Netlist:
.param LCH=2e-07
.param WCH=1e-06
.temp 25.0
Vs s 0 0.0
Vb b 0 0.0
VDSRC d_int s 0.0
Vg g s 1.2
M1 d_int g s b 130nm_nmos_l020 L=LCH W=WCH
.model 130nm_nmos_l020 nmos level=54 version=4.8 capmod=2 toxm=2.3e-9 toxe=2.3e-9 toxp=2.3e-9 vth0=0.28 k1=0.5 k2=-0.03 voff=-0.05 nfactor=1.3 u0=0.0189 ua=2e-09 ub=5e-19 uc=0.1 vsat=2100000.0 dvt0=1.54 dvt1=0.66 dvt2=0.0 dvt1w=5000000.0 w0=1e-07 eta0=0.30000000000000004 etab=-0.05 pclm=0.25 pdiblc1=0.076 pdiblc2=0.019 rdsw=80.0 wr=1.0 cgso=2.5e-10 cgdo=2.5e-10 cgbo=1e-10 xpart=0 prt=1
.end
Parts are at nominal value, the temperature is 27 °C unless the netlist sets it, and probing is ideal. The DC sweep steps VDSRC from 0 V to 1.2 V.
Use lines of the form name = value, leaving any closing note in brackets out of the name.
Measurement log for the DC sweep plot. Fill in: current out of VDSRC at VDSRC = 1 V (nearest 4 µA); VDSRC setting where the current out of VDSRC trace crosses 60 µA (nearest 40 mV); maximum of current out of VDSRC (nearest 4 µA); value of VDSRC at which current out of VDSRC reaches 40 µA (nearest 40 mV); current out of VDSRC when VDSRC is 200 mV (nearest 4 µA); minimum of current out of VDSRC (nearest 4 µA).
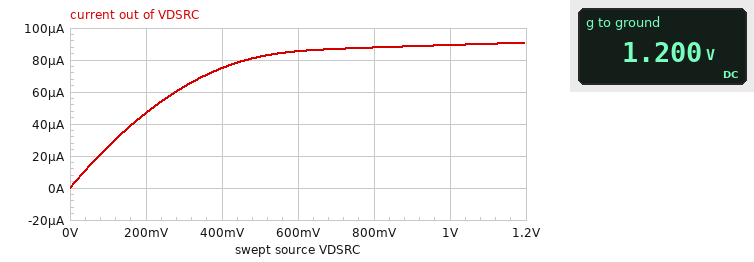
current out of VDSRC at VDSRC = 1 V = 88 µA
VDSRC setting where the current out of VDSRC trace crosses 60 µA = 280 mV
maximum of current out of VDSRC = 92 µA
value of VDSRC at which current out of VDSRC reaches 40 µA = 160 mV
current out of VDSRC when VDSRC is 200 mV = 48 µA
minimum of current out of VDSRC = 0 A
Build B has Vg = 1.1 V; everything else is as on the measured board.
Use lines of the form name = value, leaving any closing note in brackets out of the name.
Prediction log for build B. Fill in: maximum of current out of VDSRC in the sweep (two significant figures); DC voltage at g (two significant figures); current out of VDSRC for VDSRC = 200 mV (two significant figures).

maximum of current out of VDSRC in the sweep = 69 µA
DC voltage at g = 1.1 V
current out of VDSRC for VDSRC = 200 mV = 39 µA
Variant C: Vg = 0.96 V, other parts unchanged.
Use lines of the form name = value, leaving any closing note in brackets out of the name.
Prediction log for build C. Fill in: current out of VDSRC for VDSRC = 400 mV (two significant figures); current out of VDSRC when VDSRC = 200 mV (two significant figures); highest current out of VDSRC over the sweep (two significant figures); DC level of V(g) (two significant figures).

current out of VDSRC for VDSRC = 400 mV = 37 µA
current out of VDSRC when VDSRC = 200 mV = 28 µA
highest current out of VDSRC over the sweep = 41 µA
DC level of V(g) = 960 mV
